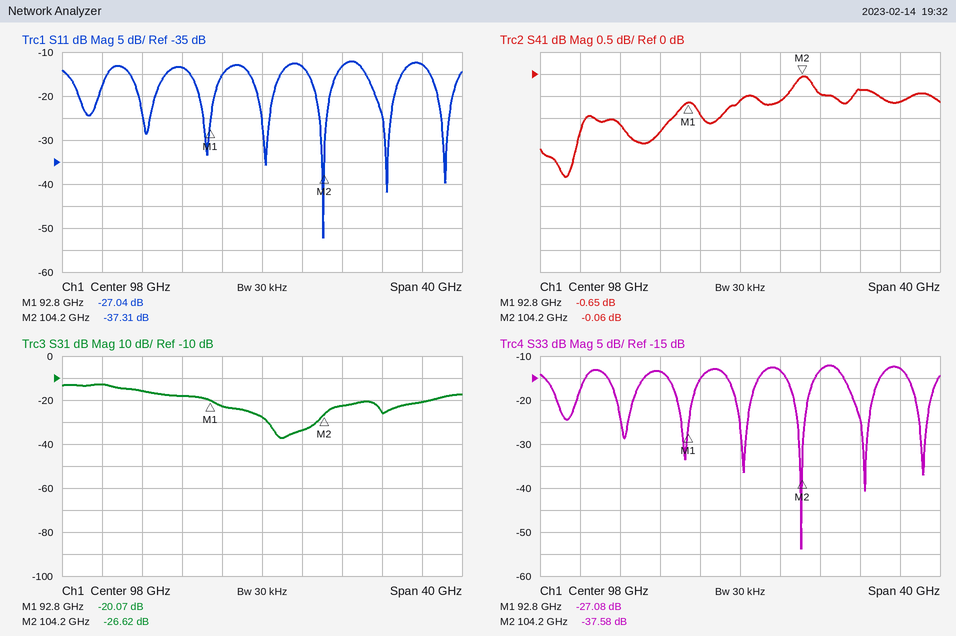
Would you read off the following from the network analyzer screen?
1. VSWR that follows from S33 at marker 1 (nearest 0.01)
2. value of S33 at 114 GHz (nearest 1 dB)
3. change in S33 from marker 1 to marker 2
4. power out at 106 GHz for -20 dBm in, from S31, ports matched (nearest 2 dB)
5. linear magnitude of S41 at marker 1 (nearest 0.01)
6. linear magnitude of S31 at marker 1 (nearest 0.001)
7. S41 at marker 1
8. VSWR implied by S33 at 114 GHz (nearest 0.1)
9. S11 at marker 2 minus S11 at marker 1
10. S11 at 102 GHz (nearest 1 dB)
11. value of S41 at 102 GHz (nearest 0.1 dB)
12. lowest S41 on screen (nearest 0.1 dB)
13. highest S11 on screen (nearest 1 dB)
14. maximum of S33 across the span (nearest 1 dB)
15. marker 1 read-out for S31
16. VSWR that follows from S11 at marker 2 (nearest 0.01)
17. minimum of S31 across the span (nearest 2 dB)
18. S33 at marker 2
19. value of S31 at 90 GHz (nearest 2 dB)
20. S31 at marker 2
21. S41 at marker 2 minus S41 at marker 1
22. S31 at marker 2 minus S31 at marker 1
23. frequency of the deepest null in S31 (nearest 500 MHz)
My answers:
1.09
-13 dB
-10.50 dB
-42 dBm
0.93
0.099
-0.65 dB
1.6
-10.27 dB
-13 dB
-0.6 dB
-2.3 dB
-12 dB
-12 dB
-20.07 dB
1.03
-38 dB
-37.58 dB
-18 dB
-26.62 dB
0.59 dB
-6.55 dB
100.0 GHz
